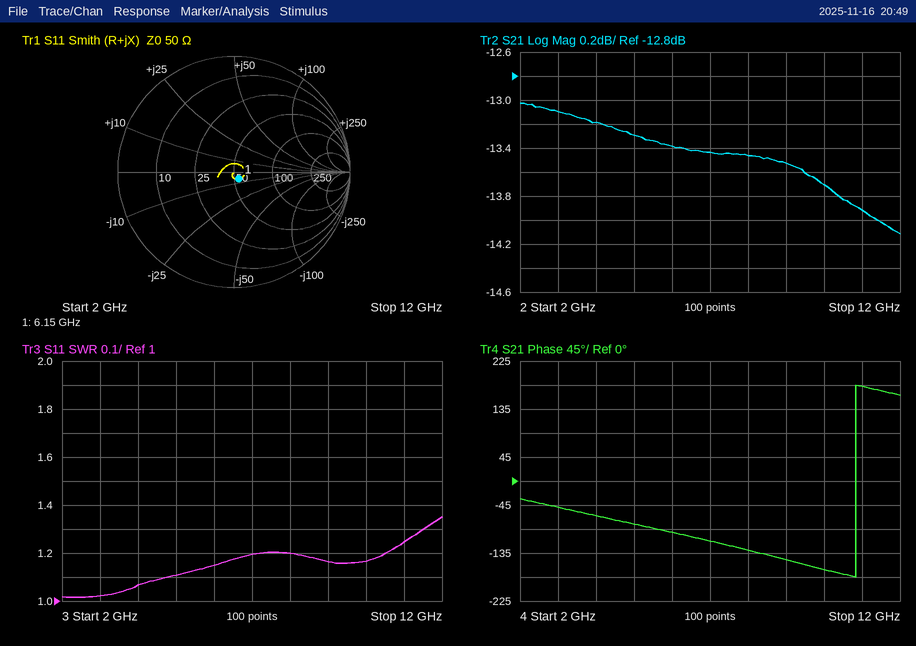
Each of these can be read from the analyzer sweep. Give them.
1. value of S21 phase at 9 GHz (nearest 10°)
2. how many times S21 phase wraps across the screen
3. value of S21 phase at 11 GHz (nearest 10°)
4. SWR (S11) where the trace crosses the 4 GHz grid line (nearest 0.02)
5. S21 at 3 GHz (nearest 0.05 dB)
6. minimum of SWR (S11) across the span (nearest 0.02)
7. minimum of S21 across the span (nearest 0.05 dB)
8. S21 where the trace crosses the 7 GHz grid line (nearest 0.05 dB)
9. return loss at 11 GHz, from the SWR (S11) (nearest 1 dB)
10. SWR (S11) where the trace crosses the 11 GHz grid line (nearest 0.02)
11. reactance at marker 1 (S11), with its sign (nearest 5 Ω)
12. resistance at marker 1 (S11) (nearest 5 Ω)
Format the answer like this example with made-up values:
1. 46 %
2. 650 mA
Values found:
1. -150°
2. 1
3. 180°
4. 1.06
5. -13.10 dB
6. 1.02
7. -14.10 dB
8. -13.45 dB
9. 19 dB
10. 1.24
11. -5 Ω
12. 55 Ω
